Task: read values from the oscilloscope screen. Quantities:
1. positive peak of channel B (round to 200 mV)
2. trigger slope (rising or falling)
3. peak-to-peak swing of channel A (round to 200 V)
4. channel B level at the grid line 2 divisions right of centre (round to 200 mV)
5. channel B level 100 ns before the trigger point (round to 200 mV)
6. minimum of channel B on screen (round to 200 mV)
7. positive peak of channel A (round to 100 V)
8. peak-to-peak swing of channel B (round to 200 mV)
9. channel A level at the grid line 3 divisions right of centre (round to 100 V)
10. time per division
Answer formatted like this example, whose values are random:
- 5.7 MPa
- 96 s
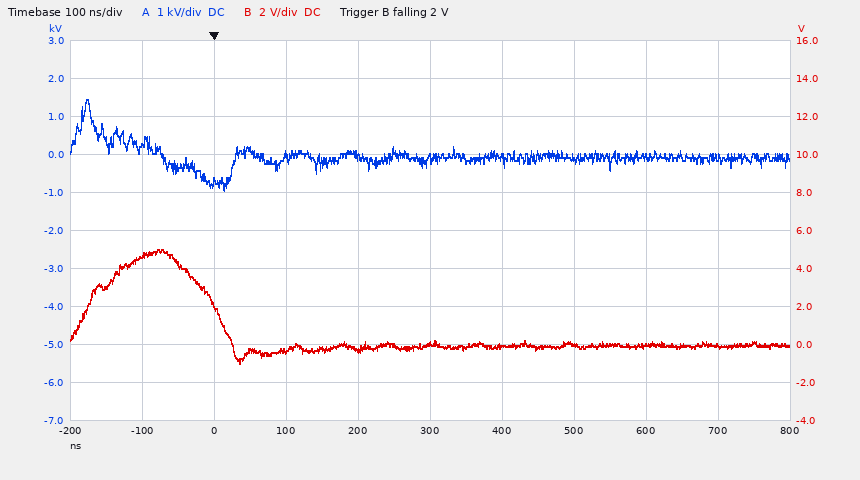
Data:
- 5.0 V
- falling
- 2.4 kV
- 0.0 V
- 4.6 V
- -1.0 V
- 1.4 kV
- 6.0 V
- -100 V
- 100 ns
